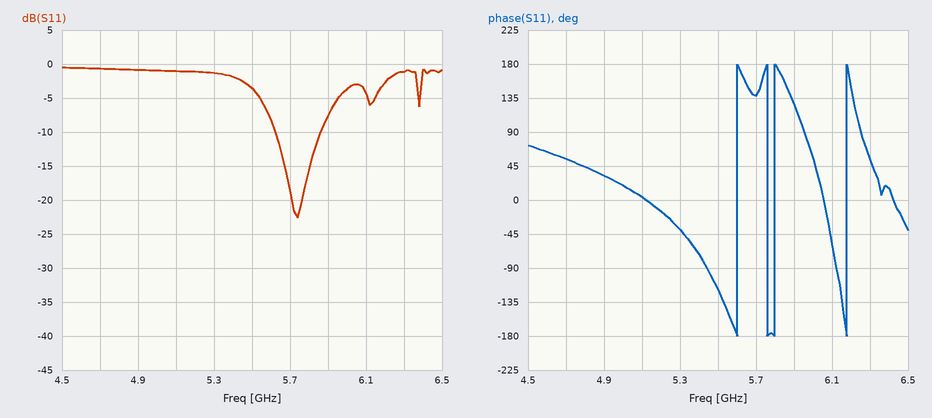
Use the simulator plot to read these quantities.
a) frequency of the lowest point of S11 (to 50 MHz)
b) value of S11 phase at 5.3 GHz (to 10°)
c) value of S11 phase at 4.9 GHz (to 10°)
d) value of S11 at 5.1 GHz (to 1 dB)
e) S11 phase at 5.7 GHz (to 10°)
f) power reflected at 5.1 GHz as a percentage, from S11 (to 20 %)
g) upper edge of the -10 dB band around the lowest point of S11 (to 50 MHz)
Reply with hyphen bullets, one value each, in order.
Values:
- 5.75 GHz
- -40°
- 30°
- -1 dB
- 140°
- 80 %
- 5.85 GHz
